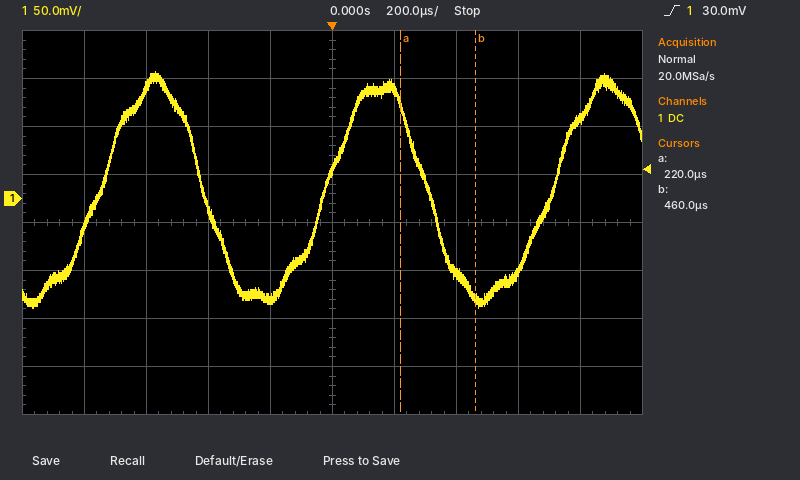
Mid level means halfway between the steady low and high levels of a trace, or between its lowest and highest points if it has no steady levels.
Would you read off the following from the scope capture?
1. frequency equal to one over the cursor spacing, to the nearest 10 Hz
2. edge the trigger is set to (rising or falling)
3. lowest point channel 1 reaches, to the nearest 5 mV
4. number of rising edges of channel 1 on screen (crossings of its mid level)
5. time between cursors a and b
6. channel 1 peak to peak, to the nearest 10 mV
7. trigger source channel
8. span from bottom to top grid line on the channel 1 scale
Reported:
4.17 kHz
rising
-115 mV
3
240 µs
250 mV
channel 1
400 mV
